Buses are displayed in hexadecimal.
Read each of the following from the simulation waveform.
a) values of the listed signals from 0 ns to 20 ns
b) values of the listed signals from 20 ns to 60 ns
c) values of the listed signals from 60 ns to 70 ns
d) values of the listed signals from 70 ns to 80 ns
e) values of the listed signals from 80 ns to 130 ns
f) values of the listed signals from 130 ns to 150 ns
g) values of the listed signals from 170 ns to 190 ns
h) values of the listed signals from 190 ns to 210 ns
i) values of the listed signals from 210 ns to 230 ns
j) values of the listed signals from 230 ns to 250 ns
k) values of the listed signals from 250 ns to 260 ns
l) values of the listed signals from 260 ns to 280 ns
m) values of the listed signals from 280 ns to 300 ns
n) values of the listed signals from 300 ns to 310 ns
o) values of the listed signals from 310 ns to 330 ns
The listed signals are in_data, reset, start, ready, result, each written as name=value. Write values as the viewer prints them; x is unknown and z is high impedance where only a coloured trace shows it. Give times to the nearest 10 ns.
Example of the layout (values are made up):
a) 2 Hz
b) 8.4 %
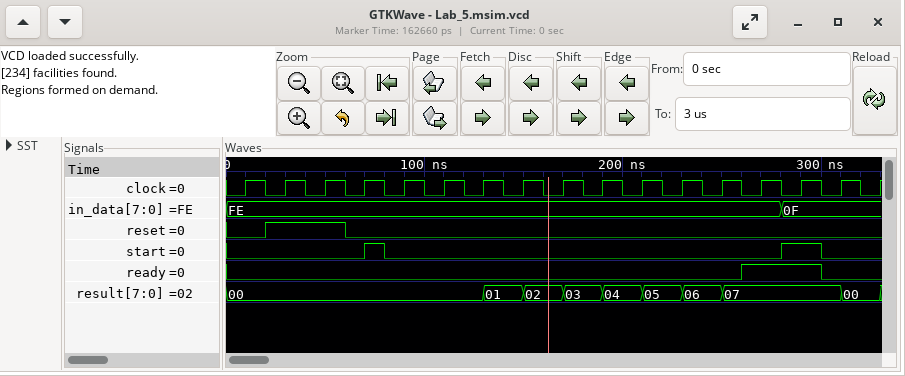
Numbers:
a) in_data=FE, reset=0, start=0, ready=0, result=00
b) in_data=FE, reset=1, start=0, ready=0, result=00
c) in_data=FE, reset=0, start=0, ready=0, result=00
d) in_data=FE, reset=0, start=1, ready=0, result=00
e) in_data=FE, reset=0, start=0, ready=0, result=00
f) in_data=FE, reset=0, start=0, ready=0, result=01
g) in_data=FE, reset=0, start=0, ready=0, result=03
h) in_data=FE, reset=0, start=0, ready=0, result=04
i) in_data=FE, reset=0, start=0, ready=0, result=05
j) in_data=FE, reset=0, start=0, ready=0, result=06
k) in_data=FE, reset=0, start=0, ready=0, result=07
l) in_data=FE, reset=0, start=0, ready=1, result=07
m) in_data=0F, reset=0, start=1, ready=1, result=07
n) in_data=0F, reset=0, start=0, ready=0, result=07
o) in_data=0F, reset=0, start=0, ready=0, result=00
